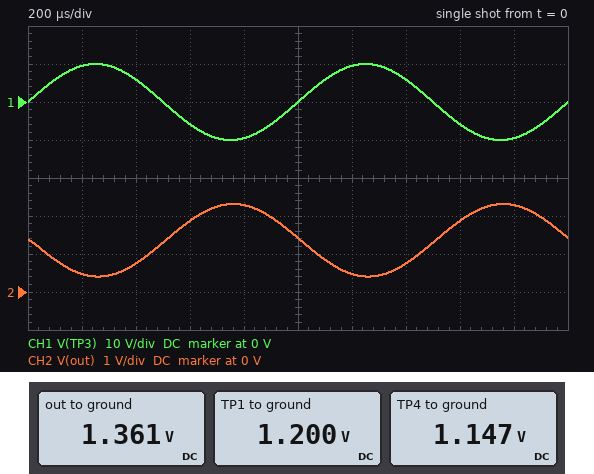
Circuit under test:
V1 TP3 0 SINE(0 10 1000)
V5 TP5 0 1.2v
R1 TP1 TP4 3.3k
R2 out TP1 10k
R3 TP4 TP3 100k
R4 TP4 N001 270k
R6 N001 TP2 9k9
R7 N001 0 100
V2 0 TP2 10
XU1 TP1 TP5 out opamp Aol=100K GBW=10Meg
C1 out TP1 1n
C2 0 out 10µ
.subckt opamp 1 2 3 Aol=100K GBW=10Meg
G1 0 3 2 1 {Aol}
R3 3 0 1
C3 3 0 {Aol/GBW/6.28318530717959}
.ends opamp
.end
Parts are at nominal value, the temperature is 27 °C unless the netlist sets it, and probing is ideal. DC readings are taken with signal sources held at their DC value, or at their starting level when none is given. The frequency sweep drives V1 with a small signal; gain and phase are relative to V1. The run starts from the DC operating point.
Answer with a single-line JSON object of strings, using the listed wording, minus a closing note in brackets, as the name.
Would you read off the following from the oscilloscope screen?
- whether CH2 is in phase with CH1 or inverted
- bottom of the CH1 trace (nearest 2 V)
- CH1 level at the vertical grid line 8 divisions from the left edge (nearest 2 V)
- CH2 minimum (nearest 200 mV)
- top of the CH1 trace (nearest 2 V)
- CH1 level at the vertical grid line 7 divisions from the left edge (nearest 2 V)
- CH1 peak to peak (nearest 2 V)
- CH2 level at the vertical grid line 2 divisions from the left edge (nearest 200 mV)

{"whether CH2 is in phase with CH1 or inverted": "inverted", "bottom of the CH1 trace": "-10 V", "CH1 level at the vertical grid line 8 divisions from the left edge": "-6 V", "CH2 minimum": "400 mV", "top of the CH1 trace": "10 V", "CH1 level at the vertical grid line 7 divisions from the left edge": "6 V", "CH1 peak to peak": "20 V", "CH2 level at the vertical grid line 2 divisions from the left edge": "800 mV"}
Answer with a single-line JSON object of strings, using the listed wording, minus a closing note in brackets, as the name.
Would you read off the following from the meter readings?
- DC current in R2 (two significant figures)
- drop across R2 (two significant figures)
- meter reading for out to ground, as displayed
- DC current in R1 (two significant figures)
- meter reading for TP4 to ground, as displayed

{"DC current in R2": "16 µA", "drop across R2": "160 mV", "meter reading for out to ground, as displayed": "1.361 V", "DC current in R1": "16 µA", "meter reading for TP4 to ground, as displayed": "1.147 V"}
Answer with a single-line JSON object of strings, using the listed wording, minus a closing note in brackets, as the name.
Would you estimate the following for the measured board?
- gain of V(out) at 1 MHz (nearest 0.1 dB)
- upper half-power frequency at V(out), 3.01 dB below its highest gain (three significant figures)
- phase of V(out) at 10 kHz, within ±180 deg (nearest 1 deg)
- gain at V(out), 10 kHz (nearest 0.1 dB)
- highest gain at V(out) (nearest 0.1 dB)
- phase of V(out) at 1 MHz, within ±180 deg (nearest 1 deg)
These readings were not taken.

{"gain of V(out) at 1 MHz": "-56.4 dB", "upper half-power frequency at V(out), 3.01 dB below its highest gain": "15.9 kHz", "phase of V(out) at 10 kHz, within ±180 deg": "148 deg", "gain at V(out), 10 kHz": "-21.8 dB", "highest gain at V(out)": "-20.4 dB", "phase of V(out) at 1 MHz, within ±180 deg": "85 deg"}
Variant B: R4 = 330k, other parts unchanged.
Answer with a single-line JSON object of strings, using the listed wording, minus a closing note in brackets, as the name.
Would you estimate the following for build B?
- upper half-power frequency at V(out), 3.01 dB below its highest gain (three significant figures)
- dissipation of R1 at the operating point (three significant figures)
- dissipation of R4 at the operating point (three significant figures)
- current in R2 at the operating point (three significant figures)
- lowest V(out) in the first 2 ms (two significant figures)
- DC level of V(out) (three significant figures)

{"upper half-power frequency at V(out), 3.01 dB below its highest gain": "15.9 kHz", "dissipation of R1 at the operating point": "771 nW", "dissipation of R4 at the operating point": "4.73 µW", "current in R2 at the operating point": "15.3 µA", "lowest V(out) in the first 2 ms": "400 mV", "DC level of V(out)": "1.35 V"}
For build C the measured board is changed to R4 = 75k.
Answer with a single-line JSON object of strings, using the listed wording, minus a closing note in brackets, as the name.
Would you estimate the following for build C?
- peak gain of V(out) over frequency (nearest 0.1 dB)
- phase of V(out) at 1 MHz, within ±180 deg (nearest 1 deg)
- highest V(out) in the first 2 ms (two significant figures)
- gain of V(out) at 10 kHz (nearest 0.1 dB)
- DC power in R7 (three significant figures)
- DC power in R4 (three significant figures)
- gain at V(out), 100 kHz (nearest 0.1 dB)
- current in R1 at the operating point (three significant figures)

{"peak gain of V(out) over frequency": "-20.6 dB", "phase of V(out) at 1 MHz, within ±180 deg": "85 deg", "highest V(out) in the first 2 ms": "2.4 V", "gain of V(out) at 10 kHz": "-22.1 dB", "DC power in R7": "96.8 µW", "DC power in R4": "19.5 µW", "gain at V(out), 100 kHz": "-36.7 dB", "current in R1 at the operating point": "27.2 µA"}
